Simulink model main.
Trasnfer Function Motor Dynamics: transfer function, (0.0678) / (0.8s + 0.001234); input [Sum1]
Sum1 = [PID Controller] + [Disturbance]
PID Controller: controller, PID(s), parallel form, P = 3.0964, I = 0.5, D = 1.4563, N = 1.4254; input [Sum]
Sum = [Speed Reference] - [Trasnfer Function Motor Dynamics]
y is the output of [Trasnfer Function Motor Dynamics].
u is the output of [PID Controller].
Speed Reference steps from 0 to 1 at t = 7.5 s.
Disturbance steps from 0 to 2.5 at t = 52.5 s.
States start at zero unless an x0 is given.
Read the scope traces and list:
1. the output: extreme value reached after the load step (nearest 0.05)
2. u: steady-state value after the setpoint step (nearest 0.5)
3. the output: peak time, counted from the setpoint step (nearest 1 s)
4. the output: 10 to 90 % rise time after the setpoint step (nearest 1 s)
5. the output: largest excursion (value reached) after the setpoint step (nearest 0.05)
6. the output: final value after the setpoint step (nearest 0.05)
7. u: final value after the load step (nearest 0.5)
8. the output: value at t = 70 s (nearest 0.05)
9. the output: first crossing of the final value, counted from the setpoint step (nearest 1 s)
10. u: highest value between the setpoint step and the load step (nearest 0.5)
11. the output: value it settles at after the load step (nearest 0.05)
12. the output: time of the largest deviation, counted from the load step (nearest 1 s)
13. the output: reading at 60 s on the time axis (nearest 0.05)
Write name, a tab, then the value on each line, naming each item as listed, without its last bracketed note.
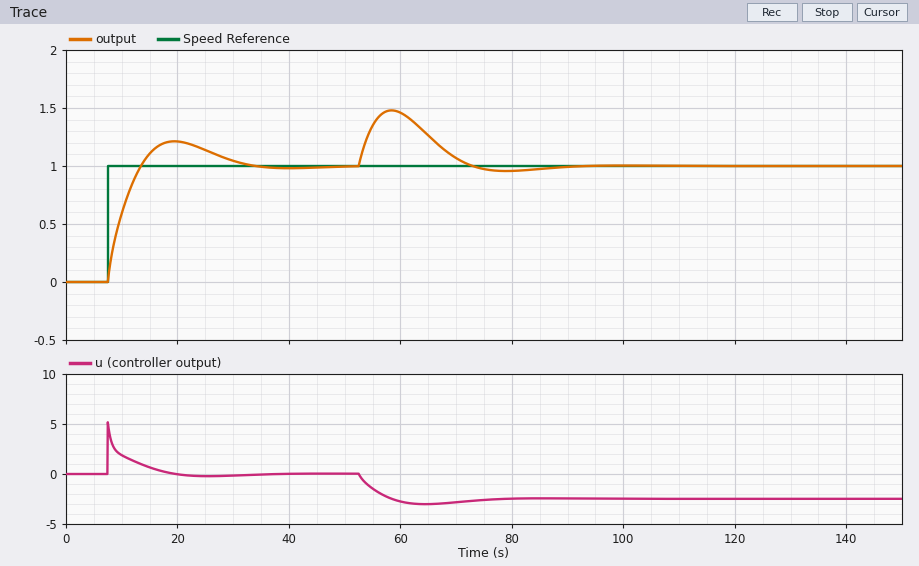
the output: extreme value reached after the load step	1.50
u: steady-state value after the setpoint step	0.0
the output: peak time, counted from the setpoint step	12 s
the output: 10 to 90 % rise time after the setpoint step	5 s
the output: largest excursion (value reached) after the setpoint step	1.20
the output: final value after the setpoint step	1.00
u: final value after the load step	-2.5
the output: value at t = 70 s	1.05
the output: first crossing of the final value, counted from the setpoint step	6 s
u: highest value between the setpoint step and the load step	5.0
the output: value it settles at after the load step	1.00
the output: time of the largest deviation, counted from the load step	6 s
the output: reading at 60 s on the time axis	1.45
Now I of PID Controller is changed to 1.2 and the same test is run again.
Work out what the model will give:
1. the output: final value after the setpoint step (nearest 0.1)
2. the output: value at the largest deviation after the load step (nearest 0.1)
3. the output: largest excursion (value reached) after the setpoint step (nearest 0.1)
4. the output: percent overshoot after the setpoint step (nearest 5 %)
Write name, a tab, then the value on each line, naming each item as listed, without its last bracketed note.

the output: final value after the setpoint step	1.0
the output: value at the largest deviation after the load step	1.4
the output: largest excursion (value reached) after the setpoint step	1.3
the output: percent overshoot after the setpoint step	30 %
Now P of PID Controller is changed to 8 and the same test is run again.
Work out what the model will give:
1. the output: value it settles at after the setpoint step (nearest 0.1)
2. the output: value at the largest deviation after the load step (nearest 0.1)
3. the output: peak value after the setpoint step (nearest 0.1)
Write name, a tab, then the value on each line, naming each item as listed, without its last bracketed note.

the output: value it settles at after the setpoint step	1.0
the output: value at the largest deviation after the load step	1.3
the output: peak value after the setpoint step	1.1
